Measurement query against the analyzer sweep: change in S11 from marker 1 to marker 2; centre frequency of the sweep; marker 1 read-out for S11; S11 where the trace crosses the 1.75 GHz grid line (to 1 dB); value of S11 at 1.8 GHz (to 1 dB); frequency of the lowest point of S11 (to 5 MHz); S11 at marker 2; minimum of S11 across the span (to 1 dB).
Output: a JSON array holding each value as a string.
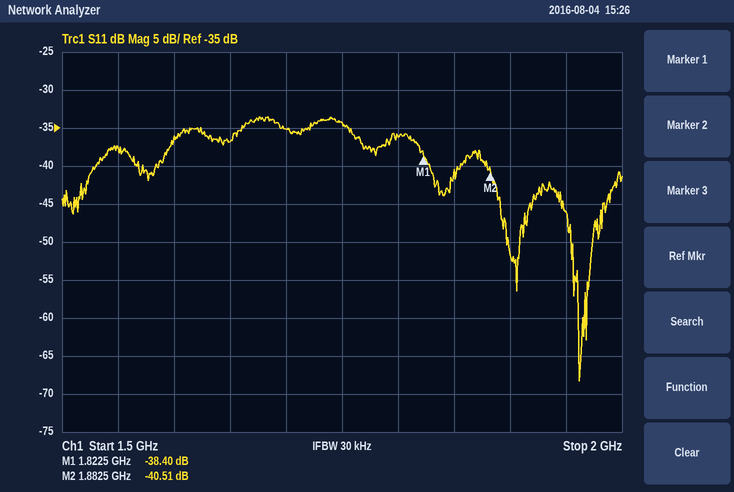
["-2.11 dB", "1.75 GHz", "-38.40 dB", "-34 dB", "-36 dB", "1.960 GHz", "-40.51 dB", "-68 dB"]
